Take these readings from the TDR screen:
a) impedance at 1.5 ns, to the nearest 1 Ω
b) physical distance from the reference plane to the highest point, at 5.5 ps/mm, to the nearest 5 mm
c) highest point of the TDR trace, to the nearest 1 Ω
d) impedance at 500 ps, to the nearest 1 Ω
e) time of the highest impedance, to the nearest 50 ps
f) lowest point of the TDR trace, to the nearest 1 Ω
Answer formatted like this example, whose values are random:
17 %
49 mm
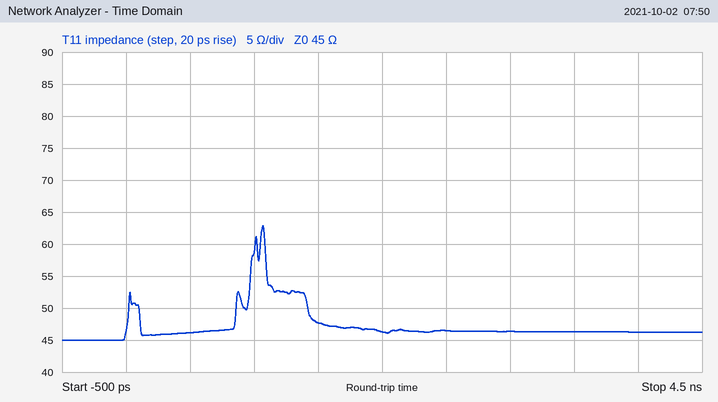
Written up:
48 Ω
95 mm
63 Ω
46 Ω
1.05 ns
45 Ω
